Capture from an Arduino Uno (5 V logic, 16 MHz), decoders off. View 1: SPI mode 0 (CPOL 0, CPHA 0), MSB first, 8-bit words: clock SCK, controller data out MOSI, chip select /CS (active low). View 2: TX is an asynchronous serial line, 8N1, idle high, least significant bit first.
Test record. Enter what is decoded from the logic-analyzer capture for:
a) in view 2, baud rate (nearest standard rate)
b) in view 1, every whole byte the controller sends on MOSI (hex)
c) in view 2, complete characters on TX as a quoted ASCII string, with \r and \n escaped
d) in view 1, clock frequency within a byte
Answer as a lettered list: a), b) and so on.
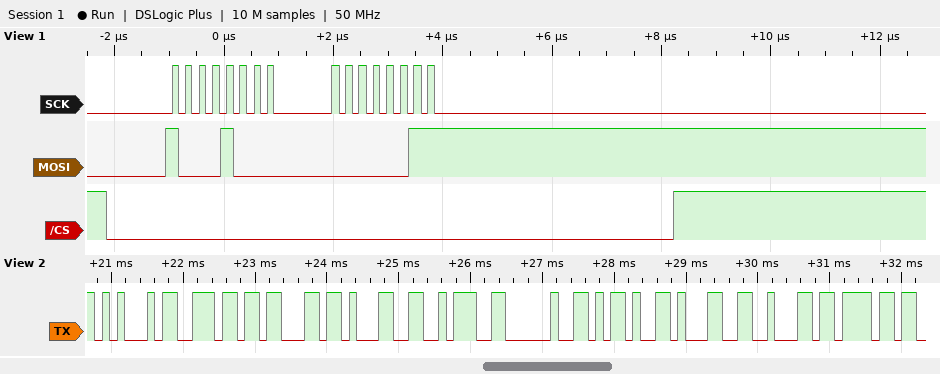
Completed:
a) 9600 baud
b) 88 03
c) "Enc1: -1bo"
d) 4 MHz
